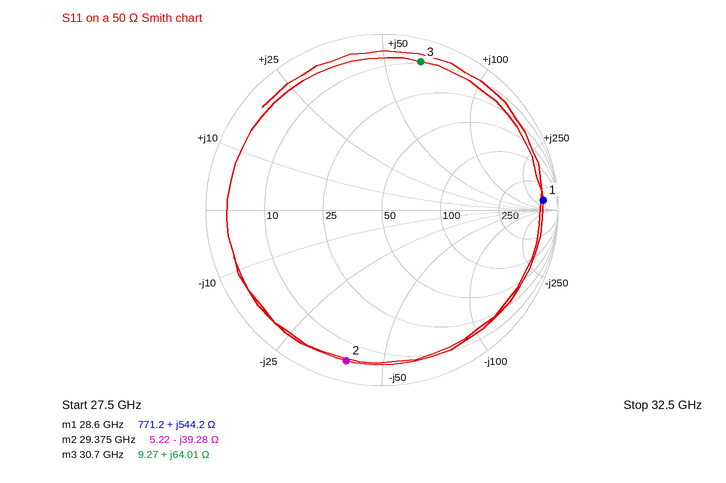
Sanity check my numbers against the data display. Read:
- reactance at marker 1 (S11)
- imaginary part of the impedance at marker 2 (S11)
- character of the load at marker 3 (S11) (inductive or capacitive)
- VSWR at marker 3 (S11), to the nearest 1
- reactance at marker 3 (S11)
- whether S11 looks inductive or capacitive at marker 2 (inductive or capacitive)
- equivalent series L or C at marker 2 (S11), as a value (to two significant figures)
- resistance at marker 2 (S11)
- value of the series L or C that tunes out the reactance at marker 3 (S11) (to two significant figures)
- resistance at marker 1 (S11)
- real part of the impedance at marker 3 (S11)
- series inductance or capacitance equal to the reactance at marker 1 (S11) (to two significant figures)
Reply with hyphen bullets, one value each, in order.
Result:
- +544.2 Ω
- -39.28 Ω
- inductive
- 14
- +64.01 Ω
- capacitive
- 140 fF
- 5.22 Ω
- 81 fF
- 771.2 Ω
- 9.27 Ω
- 3.0 nH
